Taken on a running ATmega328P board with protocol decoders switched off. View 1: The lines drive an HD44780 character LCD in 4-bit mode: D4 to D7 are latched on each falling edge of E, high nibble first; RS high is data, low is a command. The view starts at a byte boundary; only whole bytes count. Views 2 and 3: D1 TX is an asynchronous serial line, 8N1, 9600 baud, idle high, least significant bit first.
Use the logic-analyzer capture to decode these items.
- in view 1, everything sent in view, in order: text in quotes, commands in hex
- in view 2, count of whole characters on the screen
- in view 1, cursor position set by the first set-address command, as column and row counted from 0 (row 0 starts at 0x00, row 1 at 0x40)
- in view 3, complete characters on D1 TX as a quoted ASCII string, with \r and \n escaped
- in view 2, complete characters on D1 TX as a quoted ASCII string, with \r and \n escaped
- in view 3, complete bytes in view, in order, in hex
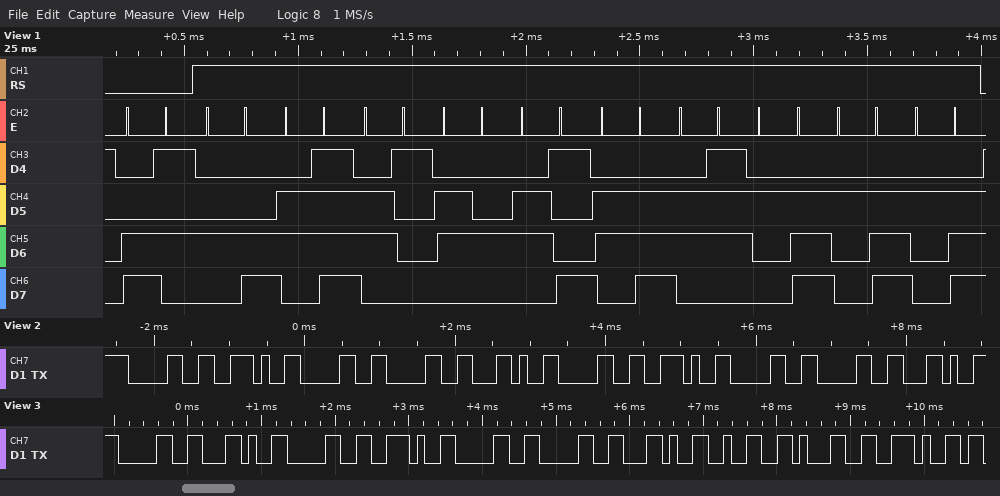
0xC5 "Loading..."
10
column 5, row 1
"0,0.00,21."
"0.00,0.00,"
0x30 0x2C 0x30 0x2E 0x30 0x30 0x2C 0x32 0x31 0x2E
